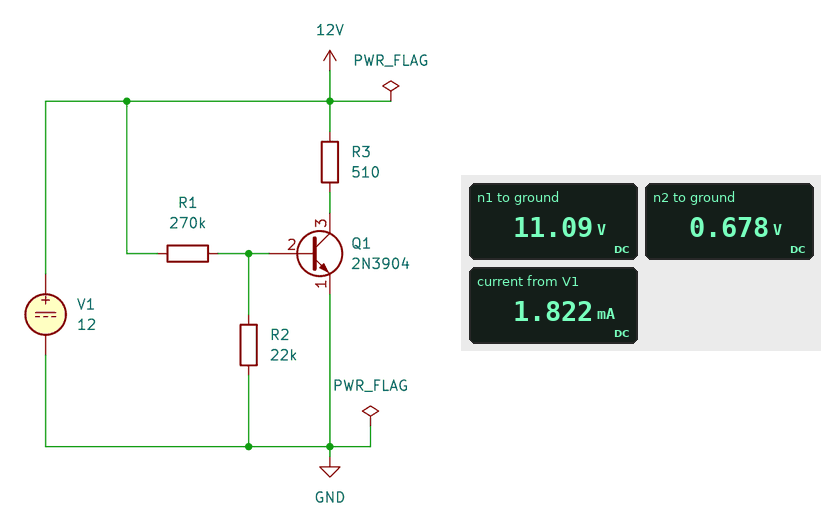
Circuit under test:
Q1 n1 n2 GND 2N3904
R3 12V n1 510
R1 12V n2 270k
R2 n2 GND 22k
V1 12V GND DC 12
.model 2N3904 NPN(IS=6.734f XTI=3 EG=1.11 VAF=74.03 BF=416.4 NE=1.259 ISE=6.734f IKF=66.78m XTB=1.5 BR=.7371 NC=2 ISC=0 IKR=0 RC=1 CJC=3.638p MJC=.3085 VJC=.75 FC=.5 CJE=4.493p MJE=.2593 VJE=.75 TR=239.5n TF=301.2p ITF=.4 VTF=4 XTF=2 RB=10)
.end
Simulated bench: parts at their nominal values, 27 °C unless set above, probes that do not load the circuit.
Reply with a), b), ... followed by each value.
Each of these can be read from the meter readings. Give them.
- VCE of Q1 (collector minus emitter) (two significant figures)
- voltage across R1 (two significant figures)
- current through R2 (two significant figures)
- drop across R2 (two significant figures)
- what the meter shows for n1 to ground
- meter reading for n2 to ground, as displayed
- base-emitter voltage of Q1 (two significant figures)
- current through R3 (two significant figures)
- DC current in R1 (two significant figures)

a) 11 V
b) 11 V
c) 31 µA
d) 680 mV
e) 11.09 V
f) 0.678 V
g) 680 mV
h) 1.8 mA
i) 42 µA
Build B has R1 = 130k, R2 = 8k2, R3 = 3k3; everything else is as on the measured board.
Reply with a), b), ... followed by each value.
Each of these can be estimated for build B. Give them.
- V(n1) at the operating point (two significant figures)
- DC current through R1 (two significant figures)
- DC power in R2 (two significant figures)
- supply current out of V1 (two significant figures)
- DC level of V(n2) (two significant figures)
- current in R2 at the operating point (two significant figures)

a) 8.9 V
b) 87 µA
c) 53 µW
d) 1.0 mA
e) 660 mV
f) 81 µA
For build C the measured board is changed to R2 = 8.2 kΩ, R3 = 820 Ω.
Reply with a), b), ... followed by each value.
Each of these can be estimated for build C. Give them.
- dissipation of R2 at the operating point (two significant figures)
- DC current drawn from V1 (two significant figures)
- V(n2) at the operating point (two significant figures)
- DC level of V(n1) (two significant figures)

a) 15 µW
b) 43 µA
c) 350 mV
d) 12 V
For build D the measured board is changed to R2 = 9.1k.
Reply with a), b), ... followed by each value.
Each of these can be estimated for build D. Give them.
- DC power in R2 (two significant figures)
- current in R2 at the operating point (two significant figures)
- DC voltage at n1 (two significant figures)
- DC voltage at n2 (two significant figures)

a) 17 µW
b) 43 µA
c) 12 V
d) 390 mV
